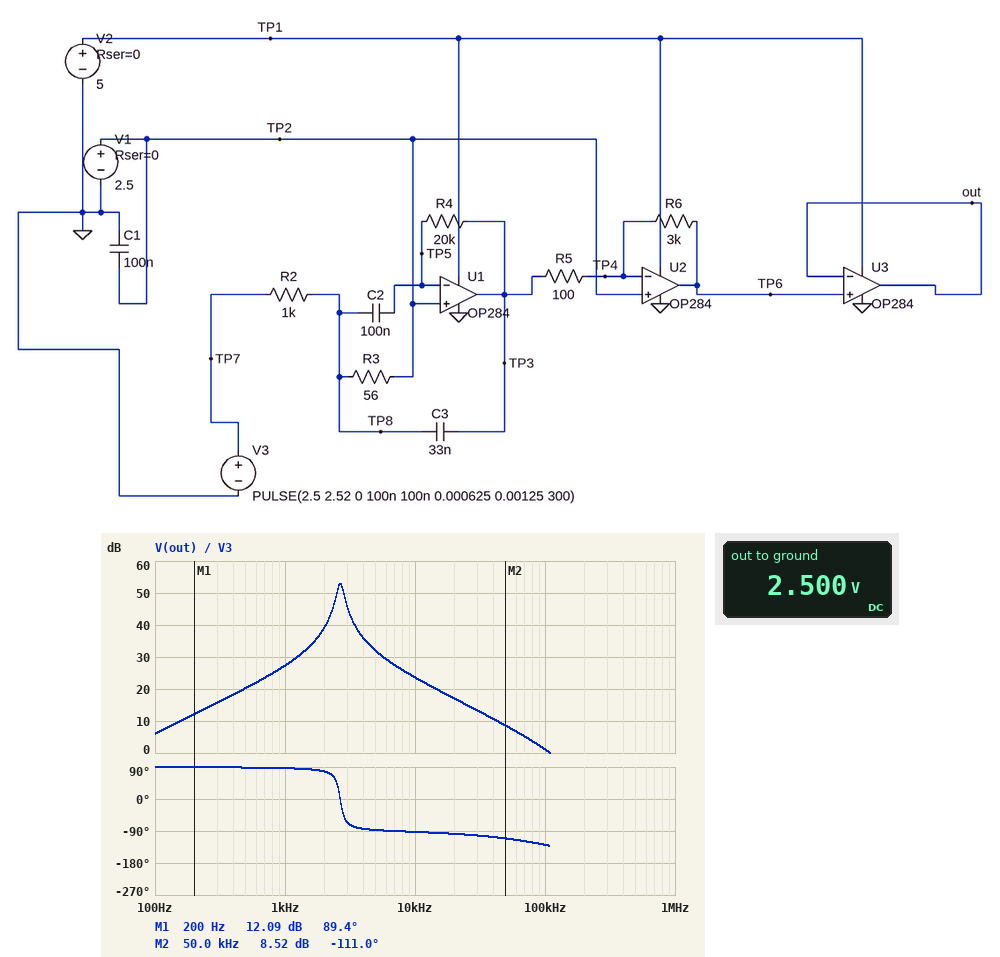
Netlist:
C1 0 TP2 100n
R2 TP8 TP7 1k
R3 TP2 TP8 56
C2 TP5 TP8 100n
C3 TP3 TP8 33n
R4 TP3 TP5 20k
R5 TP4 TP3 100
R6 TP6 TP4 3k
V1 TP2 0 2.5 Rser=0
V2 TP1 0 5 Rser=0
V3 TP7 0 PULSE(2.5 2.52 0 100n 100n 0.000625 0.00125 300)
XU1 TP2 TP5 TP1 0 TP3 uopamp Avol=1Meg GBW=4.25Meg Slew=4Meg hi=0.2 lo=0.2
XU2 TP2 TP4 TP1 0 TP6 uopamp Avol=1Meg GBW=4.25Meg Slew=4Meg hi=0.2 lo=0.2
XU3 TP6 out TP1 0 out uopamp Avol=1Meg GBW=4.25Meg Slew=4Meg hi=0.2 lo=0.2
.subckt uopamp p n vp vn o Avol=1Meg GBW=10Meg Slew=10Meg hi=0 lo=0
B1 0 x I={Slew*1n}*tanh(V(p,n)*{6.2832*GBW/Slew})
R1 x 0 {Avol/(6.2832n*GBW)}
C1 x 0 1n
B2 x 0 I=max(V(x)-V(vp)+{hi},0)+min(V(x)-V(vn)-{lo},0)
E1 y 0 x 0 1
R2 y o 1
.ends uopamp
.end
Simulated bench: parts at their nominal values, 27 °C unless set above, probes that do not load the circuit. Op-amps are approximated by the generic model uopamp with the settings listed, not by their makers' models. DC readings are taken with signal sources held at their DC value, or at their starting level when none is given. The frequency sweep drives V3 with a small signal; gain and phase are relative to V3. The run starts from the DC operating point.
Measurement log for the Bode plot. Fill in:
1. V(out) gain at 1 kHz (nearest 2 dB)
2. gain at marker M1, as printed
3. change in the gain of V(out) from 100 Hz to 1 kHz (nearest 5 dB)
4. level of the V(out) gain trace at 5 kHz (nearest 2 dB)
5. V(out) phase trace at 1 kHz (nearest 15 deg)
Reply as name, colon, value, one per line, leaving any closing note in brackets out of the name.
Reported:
V(out) gain at 1 kHz: 28 dB
gain at marker M1, as printed: 12.09 dB
change in the gain of V(out) from 100 Hz to 1 kHz: 20 dB
level of the V(out) gain trace at 5 kHz: 32 dB
V(out) phase trace at 1 kHz: 90 deg
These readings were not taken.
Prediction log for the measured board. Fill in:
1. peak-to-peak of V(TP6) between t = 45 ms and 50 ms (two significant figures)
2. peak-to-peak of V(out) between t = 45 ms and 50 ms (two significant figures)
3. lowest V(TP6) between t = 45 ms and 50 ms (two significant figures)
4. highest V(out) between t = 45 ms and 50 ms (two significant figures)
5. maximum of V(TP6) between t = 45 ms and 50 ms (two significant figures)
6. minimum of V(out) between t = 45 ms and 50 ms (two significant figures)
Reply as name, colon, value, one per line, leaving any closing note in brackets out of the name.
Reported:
peak-to-peak of V(TP6) between t = 45 ms and 50 ms: 2.4 V
peak-to-peak of V(out) between t = 45 ms and 50 ms: 2.4 V
lowest V(TP6) between t = 45 ms and 50 ms: 1.3 V
highest V(out) between t = 45 ms and 50 ms: 3.7 V
maximum of V(TP6) between t = 45 ms and 50 ms: 3.7 V
minimum of V(out) between t = 45 ms and 50 ms: 1.3 V
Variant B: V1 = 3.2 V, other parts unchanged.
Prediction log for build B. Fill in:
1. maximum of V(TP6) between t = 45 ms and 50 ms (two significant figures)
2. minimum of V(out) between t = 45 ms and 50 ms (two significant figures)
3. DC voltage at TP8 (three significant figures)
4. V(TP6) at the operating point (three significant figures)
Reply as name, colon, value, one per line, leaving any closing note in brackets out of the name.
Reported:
maximum of V(TP6) between t = 45 ms and 50 ms: 4.4 V
minimum of V(out) between t = 45 ms and 50 ms: 2.0 V
DC voltage at TP8: 3.16 V
V(TP6) at the operating point: 3.20 V
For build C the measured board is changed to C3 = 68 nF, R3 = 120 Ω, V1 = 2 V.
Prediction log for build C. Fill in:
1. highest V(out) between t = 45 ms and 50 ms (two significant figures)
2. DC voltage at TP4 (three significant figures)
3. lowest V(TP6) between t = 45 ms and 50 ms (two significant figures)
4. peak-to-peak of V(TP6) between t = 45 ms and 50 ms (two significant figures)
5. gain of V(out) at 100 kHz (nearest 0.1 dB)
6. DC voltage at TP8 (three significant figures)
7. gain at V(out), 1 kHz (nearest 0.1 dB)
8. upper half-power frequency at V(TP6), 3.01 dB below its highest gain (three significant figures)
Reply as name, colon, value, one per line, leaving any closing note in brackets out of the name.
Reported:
highest V(out) between t = 45 ms and 50 ms: 2.7 V
DC voltage at TP4: 2.00 V
lowest V(TP6) between t = 45 ms and 50 ms: 1.3 V
peak-to-peak of V(TP6) between t = 45 ms and 50 ms: 1.4 V
gain of V(out) at 100 kHz: -5.0 dB
DC voltage at TP8: 2.05 V
gain at V(out), 1 kHz: 39.3 dB
upper half-power frequency at V(TP6), 3.01 dB below its highest gain: 1.42 kHz
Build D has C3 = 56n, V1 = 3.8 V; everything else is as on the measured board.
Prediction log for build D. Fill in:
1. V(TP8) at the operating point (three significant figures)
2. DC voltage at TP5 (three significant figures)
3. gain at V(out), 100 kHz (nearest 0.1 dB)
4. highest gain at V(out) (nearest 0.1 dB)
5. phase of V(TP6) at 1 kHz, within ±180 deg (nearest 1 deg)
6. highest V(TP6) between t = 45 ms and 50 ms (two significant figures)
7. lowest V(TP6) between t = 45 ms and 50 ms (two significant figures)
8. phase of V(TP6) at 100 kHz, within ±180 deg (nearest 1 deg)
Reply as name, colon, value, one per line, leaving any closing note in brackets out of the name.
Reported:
V(TP8) at the operating point: 3.73 V
DC voltage at TP5: 3.80 V
gain at V(out), 100 kHz: -3.3 dB
highest gain at V(out): 51.7 dB
phase of V(TP6) at 1 kHz, within ±180 deg: 86 deg
highest V(TP6) between t = 45 ms and 50 ms: 4.5 V
lowest V(TP6) between t = 45 ms and 50 ms: 3.1 V
phase of V(TP6) at 100 kHz, within ±180 deg: -127 deg
